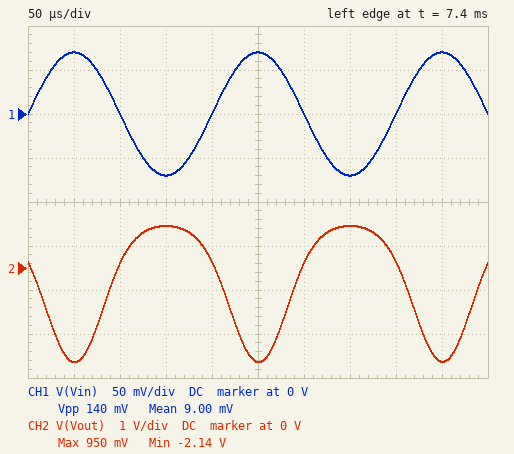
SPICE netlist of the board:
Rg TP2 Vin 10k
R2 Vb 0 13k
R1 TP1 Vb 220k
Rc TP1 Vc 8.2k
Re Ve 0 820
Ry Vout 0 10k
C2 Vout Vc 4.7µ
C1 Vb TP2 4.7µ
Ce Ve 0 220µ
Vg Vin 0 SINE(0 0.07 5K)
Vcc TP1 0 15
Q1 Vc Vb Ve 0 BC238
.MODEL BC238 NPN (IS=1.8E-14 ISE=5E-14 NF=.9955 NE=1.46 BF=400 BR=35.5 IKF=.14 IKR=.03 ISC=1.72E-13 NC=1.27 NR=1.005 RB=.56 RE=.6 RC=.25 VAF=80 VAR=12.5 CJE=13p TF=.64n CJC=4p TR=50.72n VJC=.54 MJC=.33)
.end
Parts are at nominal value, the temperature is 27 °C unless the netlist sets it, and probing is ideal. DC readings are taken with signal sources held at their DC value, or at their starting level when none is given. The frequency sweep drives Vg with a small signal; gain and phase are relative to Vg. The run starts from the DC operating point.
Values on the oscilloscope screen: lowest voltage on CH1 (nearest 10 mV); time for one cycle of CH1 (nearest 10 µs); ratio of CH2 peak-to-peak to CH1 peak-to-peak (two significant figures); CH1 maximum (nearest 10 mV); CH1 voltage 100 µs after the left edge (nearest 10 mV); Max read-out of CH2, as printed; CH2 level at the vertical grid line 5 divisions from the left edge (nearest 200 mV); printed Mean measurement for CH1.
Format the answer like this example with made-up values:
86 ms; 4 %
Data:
-70 mV; 200 µs; 22; 70 mV; 0 V; 950 mV; -2.2 V; 9.00 mV
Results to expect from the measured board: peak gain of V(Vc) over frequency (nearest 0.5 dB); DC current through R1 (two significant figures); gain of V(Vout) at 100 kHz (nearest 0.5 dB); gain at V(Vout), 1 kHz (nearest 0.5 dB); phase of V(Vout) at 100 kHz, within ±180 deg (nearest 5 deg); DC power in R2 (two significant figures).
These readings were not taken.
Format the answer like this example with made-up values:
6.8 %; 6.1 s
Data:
26.5 dB; 64 µA; 26.5 dB; 26.5 dB; 165 deg; 52 µW
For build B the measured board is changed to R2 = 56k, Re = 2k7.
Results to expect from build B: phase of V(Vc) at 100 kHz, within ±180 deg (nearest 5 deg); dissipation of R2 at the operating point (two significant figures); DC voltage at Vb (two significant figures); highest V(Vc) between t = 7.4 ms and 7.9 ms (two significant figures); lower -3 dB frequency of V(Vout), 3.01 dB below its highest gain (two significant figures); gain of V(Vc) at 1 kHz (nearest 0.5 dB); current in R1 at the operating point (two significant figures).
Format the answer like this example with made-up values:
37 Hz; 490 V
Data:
140 deg; 150 µW; 2.9 V; 11 V; 14 Hz; 35.5 dB; 55 µA
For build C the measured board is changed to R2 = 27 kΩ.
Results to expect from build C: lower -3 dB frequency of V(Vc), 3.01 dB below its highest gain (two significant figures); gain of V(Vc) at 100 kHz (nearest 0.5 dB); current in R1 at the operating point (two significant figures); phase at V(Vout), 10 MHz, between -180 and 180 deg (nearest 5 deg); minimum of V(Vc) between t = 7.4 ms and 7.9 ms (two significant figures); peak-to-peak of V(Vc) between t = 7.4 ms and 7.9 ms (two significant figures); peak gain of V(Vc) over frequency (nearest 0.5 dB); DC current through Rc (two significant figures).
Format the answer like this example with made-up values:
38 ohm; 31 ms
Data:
16 Hz; 33.5 dB; 61 µA; 85 deg; 1.2 V; 8.2 V; 36.0 dB; 1.1 mA
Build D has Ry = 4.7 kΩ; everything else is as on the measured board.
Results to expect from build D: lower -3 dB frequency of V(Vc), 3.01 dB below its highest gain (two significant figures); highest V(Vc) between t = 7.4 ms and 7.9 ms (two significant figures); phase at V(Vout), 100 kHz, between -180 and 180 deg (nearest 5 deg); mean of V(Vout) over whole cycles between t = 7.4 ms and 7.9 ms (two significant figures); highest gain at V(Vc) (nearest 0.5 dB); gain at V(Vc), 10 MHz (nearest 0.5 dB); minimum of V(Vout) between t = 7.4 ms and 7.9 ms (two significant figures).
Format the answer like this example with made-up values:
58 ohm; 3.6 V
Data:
3.3 Hz; 13 V; 170 deg; -150 mV; 23.0 dB; -3.5 dB; -1.4 V
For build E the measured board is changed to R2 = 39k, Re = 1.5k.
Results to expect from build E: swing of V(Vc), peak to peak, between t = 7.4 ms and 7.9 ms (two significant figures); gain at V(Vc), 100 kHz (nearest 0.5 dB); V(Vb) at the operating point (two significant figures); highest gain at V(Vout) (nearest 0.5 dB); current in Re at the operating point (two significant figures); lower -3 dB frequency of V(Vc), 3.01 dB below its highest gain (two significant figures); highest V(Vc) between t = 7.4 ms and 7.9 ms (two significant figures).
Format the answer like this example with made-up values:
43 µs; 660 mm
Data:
8.2 V; 33.5 dB; 2.1 V; 36.0 dB; 1.0 mA; 15 Hz; 10 V
